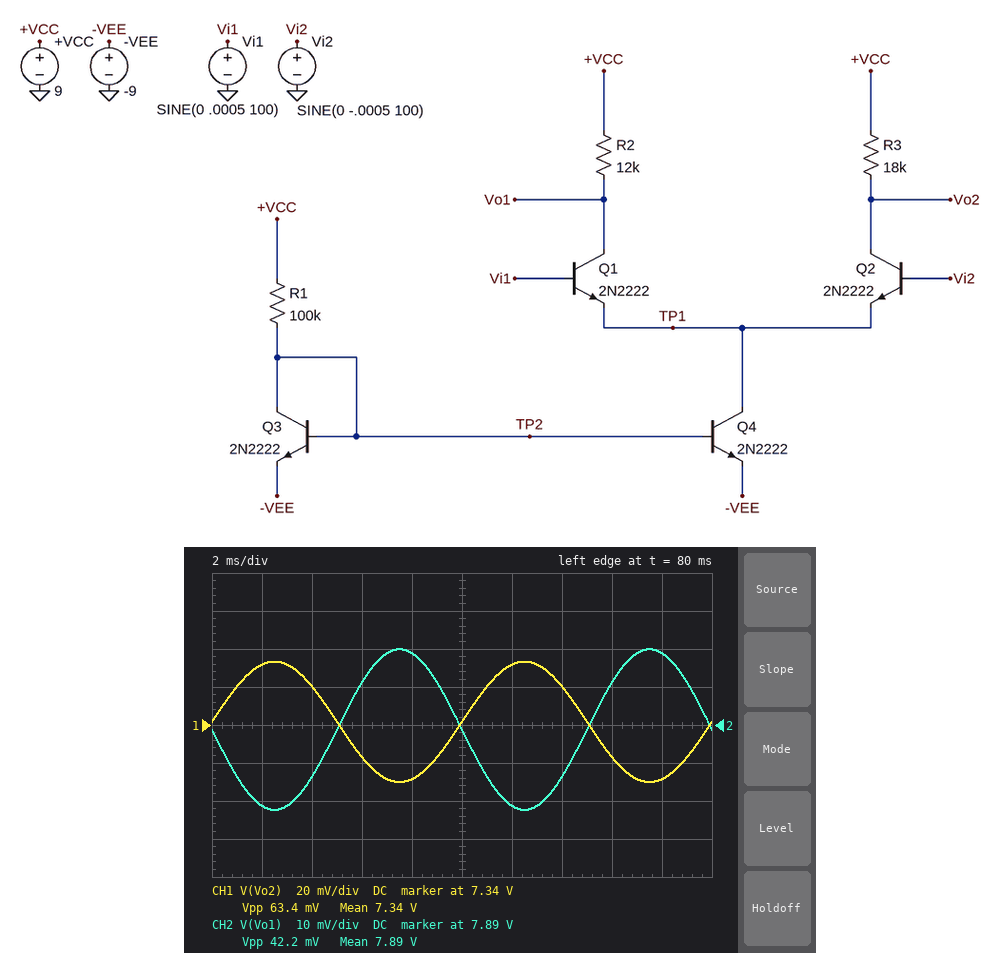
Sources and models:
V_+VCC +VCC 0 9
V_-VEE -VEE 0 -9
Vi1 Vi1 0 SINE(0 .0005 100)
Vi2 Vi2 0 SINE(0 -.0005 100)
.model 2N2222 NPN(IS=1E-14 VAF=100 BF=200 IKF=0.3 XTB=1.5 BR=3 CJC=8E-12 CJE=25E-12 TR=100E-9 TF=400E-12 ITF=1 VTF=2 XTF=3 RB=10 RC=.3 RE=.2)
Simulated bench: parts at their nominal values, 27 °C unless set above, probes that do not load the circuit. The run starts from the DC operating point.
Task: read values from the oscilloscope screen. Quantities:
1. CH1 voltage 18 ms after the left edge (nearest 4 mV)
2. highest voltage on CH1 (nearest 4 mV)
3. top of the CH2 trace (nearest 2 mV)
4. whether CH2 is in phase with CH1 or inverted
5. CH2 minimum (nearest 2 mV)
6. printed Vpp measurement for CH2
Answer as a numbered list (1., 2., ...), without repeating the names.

1. 7.312 V
2. 7.372 V
3. 7.910 V
4. inverted
5. 7.868 V
6. 42.2 mV
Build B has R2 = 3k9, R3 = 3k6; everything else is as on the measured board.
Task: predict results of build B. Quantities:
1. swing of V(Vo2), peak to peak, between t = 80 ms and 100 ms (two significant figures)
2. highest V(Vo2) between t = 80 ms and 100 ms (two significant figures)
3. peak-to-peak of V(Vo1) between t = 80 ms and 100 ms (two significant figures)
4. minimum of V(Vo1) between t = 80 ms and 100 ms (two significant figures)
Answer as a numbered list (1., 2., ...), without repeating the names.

1. 13 mV
2. 8.7 V
3. 14 mV
4. 8.6 V
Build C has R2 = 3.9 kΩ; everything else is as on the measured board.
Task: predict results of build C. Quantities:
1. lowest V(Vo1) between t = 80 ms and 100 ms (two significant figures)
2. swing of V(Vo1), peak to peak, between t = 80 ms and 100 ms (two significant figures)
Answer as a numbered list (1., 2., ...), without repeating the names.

1. 8.6 V
2. 14 mV
